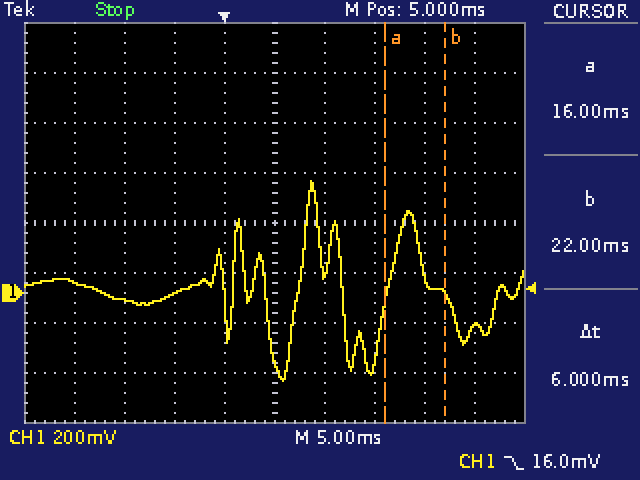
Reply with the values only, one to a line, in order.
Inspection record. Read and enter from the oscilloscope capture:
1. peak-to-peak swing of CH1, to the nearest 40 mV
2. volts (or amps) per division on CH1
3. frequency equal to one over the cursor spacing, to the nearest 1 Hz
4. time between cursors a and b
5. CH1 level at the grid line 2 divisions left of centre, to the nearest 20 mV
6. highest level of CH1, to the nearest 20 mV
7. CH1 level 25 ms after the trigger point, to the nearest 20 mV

800 mV
200 mV
167 Hz
6 ms
0 mV
440 mV
-140 mV
